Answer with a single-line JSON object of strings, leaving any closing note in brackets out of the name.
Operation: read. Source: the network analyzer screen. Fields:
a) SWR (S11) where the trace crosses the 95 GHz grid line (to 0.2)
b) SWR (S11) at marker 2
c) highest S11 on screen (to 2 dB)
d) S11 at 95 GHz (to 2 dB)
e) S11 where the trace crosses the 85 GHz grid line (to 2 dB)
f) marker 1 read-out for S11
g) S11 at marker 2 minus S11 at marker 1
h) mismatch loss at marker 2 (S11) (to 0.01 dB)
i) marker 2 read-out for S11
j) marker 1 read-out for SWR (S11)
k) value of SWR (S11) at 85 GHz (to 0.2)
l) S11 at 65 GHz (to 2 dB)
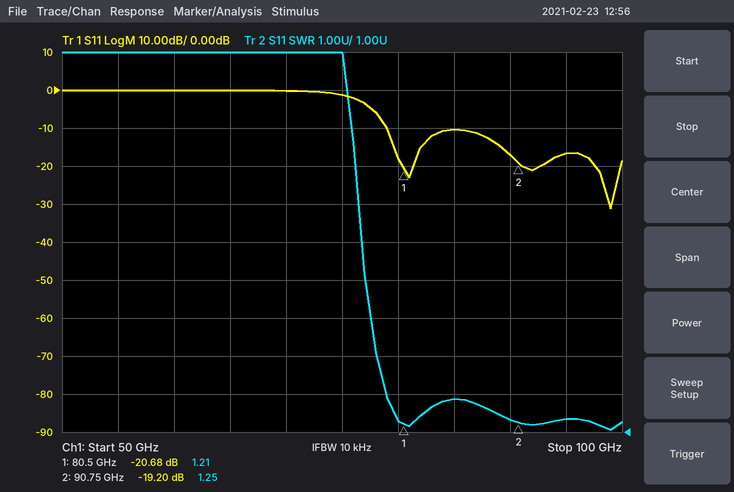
{"SWR (S11) where the trace crosses the 95 GHz grid line": "1.4", "SWR (S11) at marker 2": "1.25", "highest S11 on screen": "0 dB", "S11 at 95 GHz": "-16 dB", "S11 where the trace crosses the 85 GHz grid line": "-10 dB", "marker 1 read-out for S11": "-20.68 dB", "S11 at marker 2 minus S11 at marker 1": "1.48 dB", "mismatch loss at marker 2 (S11)": "0.05 dB", "marker 2 read-out for S11": "-19.20 dB", "marker 1 read-out for SWR": "1.21", "value of SWR (S11) at 85 GHz": "1.8", "S11 at 65 GHz": "0 dB"}
